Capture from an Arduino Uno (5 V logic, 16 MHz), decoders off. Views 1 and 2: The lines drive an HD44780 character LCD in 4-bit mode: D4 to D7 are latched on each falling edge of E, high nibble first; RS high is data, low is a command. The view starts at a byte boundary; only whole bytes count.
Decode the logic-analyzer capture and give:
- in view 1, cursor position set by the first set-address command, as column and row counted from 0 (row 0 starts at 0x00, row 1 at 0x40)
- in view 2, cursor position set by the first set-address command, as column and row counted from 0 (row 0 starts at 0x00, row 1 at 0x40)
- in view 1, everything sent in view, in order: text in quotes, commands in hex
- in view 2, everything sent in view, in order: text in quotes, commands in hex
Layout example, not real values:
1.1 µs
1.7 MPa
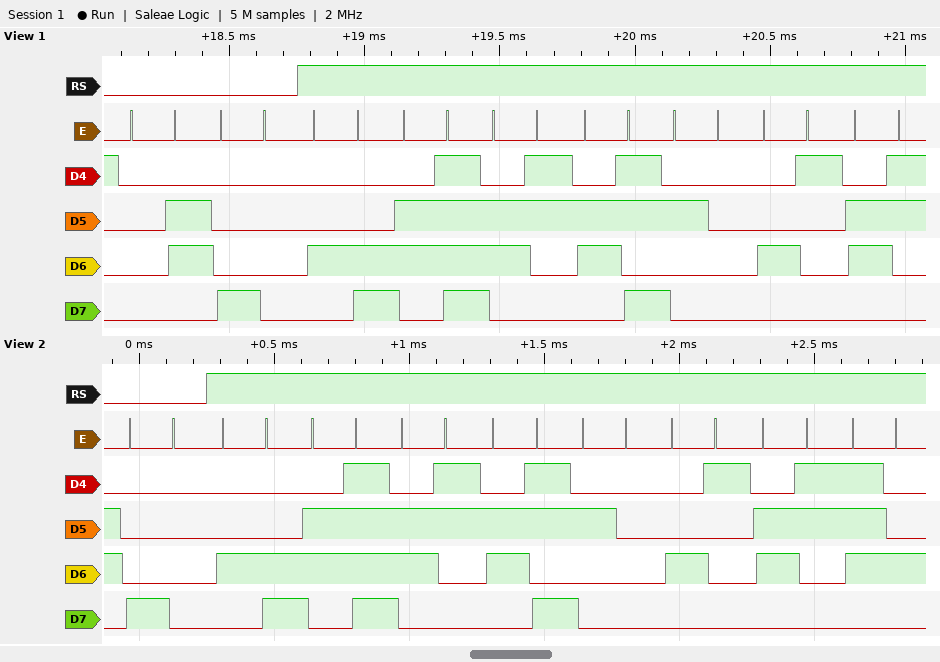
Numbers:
column 0, row 0
column 0, row 0
0x06 0x80 "Lock Ac"
0x80 "Lock Act"
